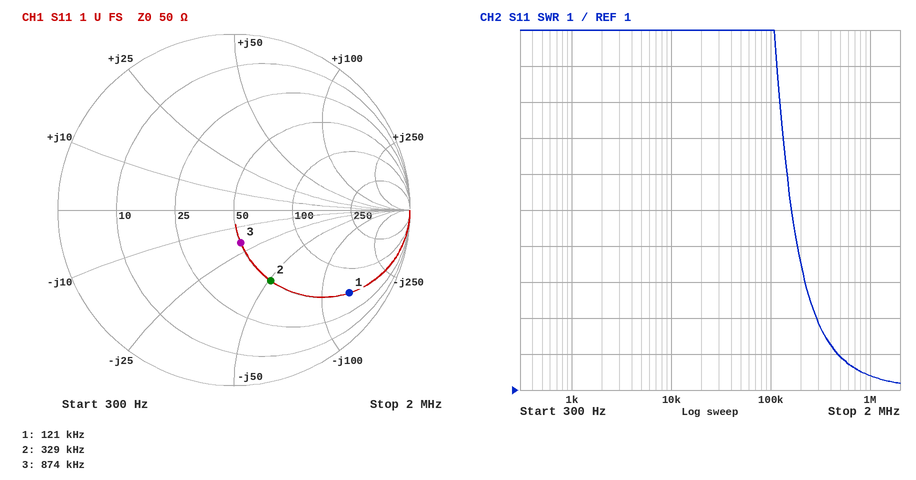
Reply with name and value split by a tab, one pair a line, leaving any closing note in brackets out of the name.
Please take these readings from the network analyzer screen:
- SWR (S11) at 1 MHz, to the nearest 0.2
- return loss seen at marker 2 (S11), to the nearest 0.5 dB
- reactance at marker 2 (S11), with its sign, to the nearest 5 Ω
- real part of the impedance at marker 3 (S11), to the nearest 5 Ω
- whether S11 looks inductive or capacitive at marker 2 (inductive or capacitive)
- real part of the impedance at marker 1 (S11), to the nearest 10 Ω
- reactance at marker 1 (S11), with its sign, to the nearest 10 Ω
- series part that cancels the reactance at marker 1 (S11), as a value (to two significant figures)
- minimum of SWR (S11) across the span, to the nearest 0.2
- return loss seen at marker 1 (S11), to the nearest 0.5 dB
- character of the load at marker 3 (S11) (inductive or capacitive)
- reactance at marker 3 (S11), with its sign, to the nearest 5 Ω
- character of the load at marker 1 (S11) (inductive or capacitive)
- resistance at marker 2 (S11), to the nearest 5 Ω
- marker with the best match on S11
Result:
SWR (S11) at 1 MHz, to the nearest 0.2	1.4
return loss seen at marker 2 (S11), to the nearest 0.5 dB	7.0 dB
reactance at marker 2 (S11), with its sign, to the nearest 5 Ω	-50 Ω
real part of the impedance at marker 3 (S11), to the nearest 5 Ω	50 Ω
whether S11 looks inductive or capacitive at marker 2	capacitive
real part of the impedance at marker 1 (S11), to the nearest 10 Ω	50 Ω
reactance at marker 1 (S11), with its sign, to the nearest 10 Ω	-140 Ω
series part that cancels the reactance at marker 1 (S11), as a value	180 µH
minimum of SWR (S11) across the span, to the nearest 0.2	1.2
return loss seen at marker 1 (S11), to the nearest 0.5 dB	2.0 dB
character of the load at marker 3 (S11)	capacitive
reactance at marker 3 (S11), with its sign, to the nearest 5 Ω	-20 Ω
character of the load at marker 1 (S11)	capacitive
resistance at marker 2 (S11), to the nearest 5 Ω	50 Ω
marker with the best match on S11	marker 3
